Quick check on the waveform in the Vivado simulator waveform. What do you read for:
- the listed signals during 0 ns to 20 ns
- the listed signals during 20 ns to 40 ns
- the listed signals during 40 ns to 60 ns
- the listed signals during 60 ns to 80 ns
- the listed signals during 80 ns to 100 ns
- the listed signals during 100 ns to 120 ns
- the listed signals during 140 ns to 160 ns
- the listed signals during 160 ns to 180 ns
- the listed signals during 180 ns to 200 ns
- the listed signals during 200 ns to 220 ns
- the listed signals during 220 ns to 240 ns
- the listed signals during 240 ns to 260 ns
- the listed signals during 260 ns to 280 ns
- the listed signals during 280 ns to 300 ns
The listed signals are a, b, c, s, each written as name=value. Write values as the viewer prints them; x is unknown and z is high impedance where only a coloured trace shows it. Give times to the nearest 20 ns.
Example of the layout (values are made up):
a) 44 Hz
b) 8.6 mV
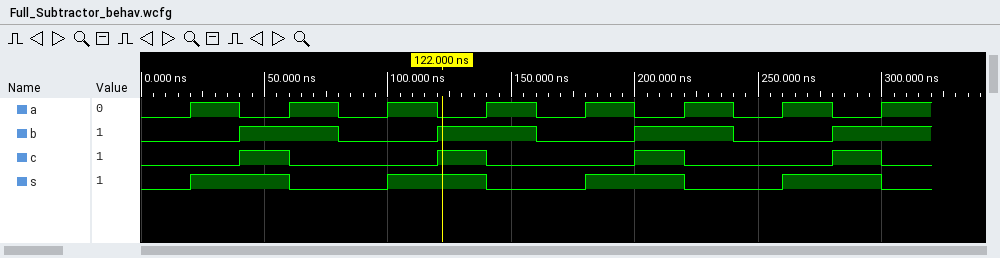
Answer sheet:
a) a=0, b=0, c=0, s=0
b) a=1, b=0, c=0, s=1
c) a=0, b=1, c=1, s=1
d) a=1, b=1, c=0, s=0
e) a=0, b=0, c=0, s=0
f) a=1, b=0, c=0, s=1
g) a=1, b=1, c=0, s=0
h) a=0, b=0, c=0, s=0
i) a=1, b=0, c=0, s=1
j) a=0, b=1, c=1, s=1
k) a=1, b=1, c=0, s=0
l) a=0, b=0, c=0, s=0
m) a=1, b=0, c=0, s=1
n) a=0, b=1, c=1, s=1
